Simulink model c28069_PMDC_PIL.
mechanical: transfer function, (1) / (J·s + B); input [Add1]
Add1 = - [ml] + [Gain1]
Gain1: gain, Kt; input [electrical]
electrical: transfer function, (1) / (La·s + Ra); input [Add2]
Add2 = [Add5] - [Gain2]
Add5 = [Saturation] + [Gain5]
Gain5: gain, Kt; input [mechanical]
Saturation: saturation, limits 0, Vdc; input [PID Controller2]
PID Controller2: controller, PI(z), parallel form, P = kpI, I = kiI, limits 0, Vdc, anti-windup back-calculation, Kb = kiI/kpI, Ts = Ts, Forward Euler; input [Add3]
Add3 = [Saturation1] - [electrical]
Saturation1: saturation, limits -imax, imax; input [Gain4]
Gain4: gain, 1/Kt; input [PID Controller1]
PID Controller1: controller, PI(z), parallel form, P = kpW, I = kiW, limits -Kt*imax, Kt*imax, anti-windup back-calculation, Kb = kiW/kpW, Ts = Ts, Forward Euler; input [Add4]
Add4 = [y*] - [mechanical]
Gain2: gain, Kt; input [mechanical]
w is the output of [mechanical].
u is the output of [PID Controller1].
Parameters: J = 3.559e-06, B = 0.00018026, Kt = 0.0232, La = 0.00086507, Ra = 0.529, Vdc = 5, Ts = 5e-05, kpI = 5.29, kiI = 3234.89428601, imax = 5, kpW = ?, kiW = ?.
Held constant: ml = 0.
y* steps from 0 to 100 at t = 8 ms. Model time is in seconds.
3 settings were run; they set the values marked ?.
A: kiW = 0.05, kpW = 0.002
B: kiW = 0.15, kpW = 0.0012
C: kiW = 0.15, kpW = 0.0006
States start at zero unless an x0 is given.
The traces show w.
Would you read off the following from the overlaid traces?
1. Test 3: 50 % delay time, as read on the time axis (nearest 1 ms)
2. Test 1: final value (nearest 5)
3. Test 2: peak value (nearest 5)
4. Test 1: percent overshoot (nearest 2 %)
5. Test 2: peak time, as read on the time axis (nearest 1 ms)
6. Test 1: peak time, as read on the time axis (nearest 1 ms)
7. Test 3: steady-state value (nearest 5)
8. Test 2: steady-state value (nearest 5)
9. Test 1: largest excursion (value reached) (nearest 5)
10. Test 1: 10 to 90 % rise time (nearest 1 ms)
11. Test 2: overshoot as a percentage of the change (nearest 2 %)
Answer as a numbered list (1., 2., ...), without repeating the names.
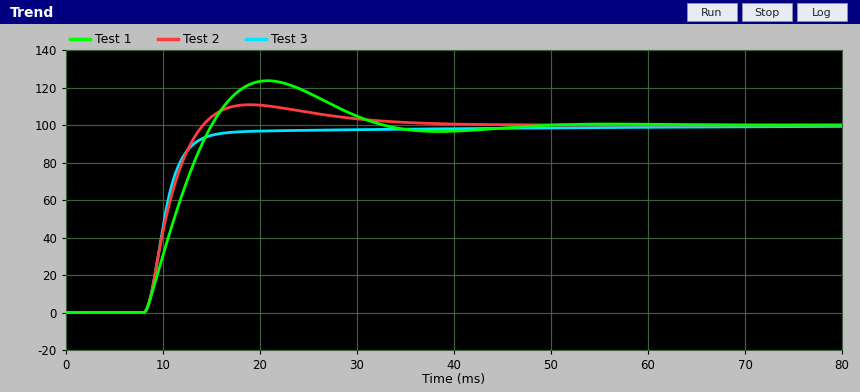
1. 10 ms
2. 100
3. 110
4. 24 %
5. 19 ms
6. 21 ms
7. 100
8. 100
9. 125
10. 5 ms
11. 10 %
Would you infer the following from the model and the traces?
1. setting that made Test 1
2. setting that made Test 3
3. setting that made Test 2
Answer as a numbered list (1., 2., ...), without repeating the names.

1. C
2. A
3. B
